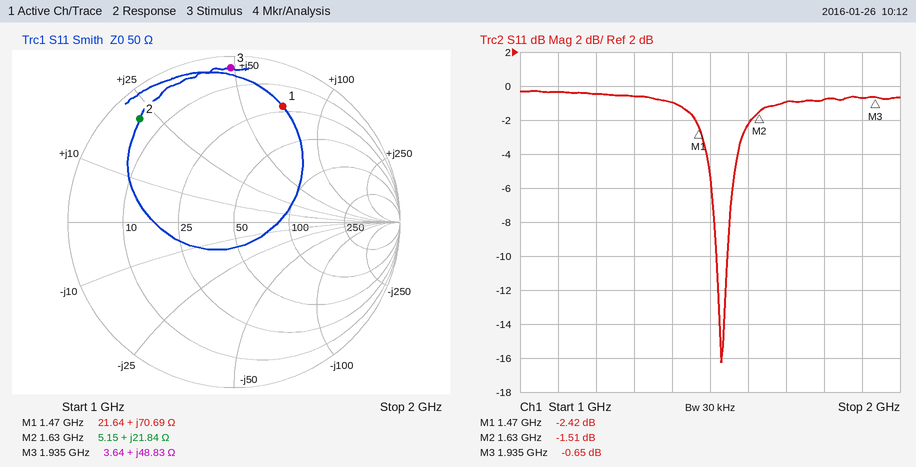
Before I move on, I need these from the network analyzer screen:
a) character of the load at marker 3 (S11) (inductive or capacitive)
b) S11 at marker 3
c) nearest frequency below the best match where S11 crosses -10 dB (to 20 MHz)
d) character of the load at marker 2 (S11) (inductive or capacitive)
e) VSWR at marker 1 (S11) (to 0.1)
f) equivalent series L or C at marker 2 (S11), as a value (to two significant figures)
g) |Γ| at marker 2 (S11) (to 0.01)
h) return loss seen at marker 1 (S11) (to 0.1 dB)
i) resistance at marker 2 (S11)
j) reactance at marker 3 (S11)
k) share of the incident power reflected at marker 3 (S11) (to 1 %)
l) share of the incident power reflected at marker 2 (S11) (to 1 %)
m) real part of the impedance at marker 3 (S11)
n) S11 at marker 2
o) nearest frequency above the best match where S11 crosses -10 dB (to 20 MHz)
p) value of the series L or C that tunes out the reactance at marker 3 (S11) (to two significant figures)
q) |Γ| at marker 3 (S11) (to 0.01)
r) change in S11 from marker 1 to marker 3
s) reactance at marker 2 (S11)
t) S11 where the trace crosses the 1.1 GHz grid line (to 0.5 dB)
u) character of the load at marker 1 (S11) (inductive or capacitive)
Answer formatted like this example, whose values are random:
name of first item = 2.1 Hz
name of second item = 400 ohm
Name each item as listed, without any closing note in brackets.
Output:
character of the load at marker 3 (S11) = inductive
S11 at marker 3 = -0.65 dB
nearest frequency below the best match where S11 crosses -10 dB = 1.52 GHz
character of the load at marker 2 (S11) = inductive
VSWR at marker 1 (S11) = 7.2
equivalent series L or C at marker 2 (S11), as a value = 2.1 nH
|Γ| at marker 2 (S11) = 0.84
return loss seen at marker 1 (S11) = 2.4 dB
resistance at marker 2 = 5.15 Ω
reactance at marker 3 = +48.83 Ω
share of the incident power reflected at marker 3 (S11) = 86 %
share of the incident power reflected at marker 2 (S11) = 71 %
real part of the impedance at marker 3 = 3.64 Ω
S11 at marker 2 = -1.51 dB
nearest frequency above the best match where S11 crosses -10 dB = 1.54 GHz
value of the series L or C that tunes out the reactance at marker 3 (S11) = 1.7 pF
|Γ| at marker 3 (S11) = 0.93
change in S11 from marker 1 to marker 3 = 1.77 dB
reactance at marker 2 = +21.84 Ω
S11 where the trace crosses the 1.1 GHz grid line = -0.5 dB
character of the load at marker 1 (S11) = inductive
